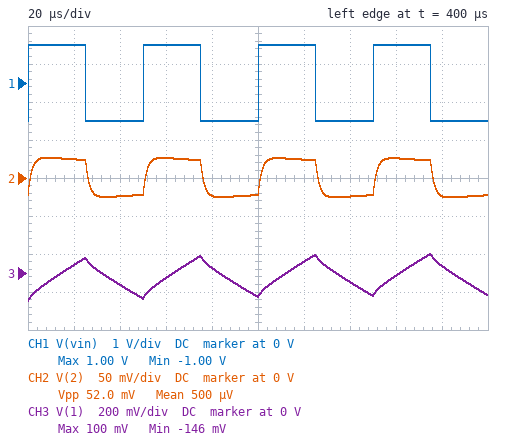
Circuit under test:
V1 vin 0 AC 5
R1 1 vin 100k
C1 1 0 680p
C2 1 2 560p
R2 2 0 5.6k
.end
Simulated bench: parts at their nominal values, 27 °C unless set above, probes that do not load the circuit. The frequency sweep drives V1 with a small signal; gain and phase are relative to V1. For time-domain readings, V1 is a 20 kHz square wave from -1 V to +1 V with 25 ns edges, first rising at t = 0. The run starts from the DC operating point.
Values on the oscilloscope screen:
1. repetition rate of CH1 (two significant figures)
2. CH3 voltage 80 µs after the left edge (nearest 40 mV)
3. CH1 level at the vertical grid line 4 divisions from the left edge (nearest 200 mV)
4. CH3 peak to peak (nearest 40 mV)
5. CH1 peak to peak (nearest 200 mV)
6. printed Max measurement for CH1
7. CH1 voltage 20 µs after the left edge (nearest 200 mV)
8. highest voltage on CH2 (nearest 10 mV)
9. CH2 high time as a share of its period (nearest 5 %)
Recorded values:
20 kHz
40 mV
-1.0 V
240 mV
2.0 V
1.00 V
1.0 V
30 mV
50 %
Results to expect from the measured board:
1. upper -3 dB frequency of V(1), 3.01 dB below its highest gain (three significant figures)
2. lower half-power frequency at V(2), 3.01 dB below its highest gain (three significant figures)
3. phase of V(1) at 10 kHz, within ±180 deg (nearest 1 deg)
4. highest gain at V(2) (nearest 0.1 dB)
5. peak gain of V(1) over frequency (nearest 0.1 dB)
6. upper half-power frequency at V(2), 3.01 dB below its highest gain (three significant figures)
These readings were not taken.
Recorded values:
1.27 kHz
1.24 kHz
-78 deg
-32.2 dB
0 dB
96.1 kHz
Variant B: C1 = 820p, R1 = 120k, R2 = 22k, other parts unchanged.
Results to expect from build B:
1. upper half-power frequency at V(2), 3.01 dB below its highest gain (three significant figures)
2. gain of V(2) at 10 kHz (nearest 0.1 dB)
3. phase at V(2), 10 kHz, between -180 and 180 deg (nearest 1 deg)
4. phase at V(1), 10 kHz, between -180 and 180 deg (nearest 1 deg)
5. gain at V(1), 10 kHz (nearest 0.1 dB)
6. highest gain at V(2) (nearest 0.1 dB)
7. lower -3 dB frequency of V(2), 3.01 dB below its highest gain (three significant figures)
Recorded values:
24.2 kHz
-23.7 dB
-19 deg
-71 deg
-19.4 dB
-23.2 dB
863 Hz
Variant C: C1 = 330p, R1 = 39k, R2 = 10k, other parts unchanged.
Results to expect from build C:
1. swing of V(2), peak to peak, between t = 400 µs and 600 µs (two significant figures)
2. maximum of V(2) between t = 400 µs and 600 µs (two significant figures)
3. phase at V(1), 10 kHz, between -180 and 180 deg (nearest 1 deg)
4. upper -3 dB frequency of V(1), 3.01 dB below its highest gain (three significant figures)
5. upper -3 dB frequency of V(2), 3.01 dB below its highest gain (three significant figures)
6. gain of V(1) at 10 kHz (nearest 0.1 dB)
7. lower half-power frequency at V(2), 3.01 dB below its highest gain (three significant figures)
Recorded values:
320 mV
160 mV
-55 deg
4.22 kHz
92.8 kHz
-7.9 dB
3.79 kHz
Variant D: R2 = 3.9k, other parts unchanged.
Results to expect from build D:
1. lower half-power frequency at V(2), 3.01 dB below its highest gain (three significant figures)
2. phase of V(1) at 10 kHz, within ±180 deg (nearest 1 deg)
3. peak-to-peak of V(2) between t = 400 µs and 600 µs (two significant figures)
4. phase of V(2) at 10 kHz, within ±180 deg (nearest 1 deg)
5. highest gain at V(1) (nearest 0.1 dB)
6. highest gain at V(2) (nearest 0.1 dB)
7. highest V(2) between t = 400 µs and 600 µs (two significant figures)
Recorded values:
1.25 kHz
-79 deg
37 mV
3 deg
0 dB
-35.2 dB
19 mV
